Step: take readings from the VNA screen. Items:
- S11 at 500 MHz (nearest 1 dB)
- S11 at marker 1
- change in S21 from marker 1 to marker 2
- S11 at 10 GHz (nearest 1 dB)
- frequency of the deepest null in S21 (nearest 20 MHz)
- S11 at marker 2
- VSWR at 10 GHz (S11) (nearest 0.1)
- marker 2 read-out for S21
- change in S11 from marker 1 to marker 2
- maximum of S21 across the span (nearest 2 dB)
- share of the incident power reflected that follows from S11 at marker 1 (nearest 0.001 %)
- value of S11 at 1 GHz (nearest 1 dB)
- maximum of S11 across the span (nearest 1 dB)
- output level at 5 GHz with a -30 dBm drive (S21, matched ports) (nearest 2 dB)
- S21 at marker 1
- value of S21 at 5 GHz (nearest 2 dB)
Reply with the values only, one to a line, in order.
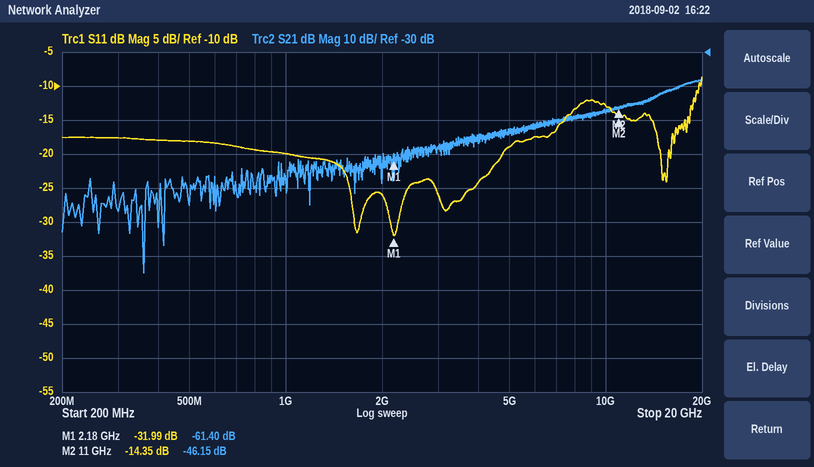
-18 dB
-31.99 dB
15.25 dB
-13 dB
360 MHz
-14.35 dB
1.6
-46.15 dB
17.64 dB
-38 dB
0.063 %
-20 dB
-9 dB
-84 dBm
-61.40 dB
-54 dB
